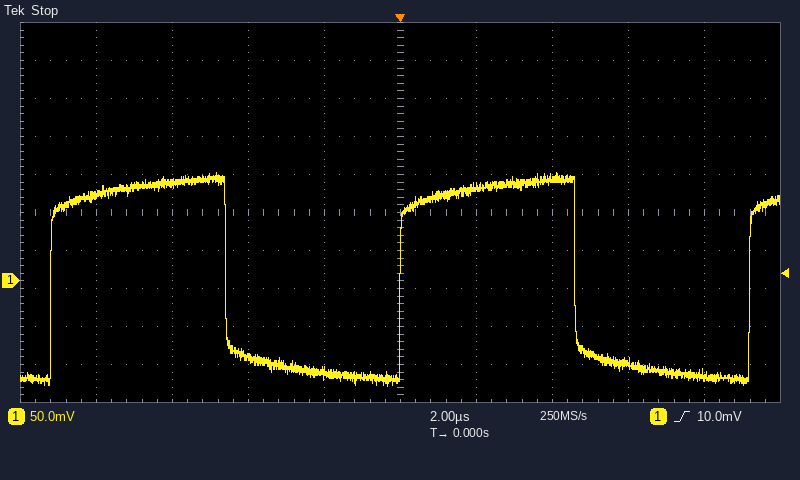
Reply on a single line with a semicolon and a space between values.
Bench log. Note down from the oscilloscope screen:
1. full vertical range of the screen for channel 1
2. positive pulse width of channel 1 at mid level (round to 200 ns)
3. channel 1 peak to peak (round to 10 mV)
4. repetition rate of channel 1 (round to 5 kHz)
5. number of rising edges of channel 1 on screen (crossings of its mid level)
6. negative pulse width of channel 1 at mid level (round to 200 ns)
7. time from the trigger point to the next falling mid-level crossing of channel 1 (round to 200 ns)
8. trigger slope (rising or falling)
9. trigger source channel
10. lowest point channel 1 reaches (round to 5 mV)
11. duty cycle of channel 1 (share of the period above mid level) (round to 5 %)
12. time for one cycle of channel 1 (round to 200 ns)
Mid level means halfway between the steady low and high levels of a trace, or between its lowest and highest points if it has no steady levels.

500 mV; 4.6 µs; 280 mV; 110 kHz; 3; 4.6 µs; 4.6 µs; rising; channel 1; -140 mV; 50 %; 9.2 µs
